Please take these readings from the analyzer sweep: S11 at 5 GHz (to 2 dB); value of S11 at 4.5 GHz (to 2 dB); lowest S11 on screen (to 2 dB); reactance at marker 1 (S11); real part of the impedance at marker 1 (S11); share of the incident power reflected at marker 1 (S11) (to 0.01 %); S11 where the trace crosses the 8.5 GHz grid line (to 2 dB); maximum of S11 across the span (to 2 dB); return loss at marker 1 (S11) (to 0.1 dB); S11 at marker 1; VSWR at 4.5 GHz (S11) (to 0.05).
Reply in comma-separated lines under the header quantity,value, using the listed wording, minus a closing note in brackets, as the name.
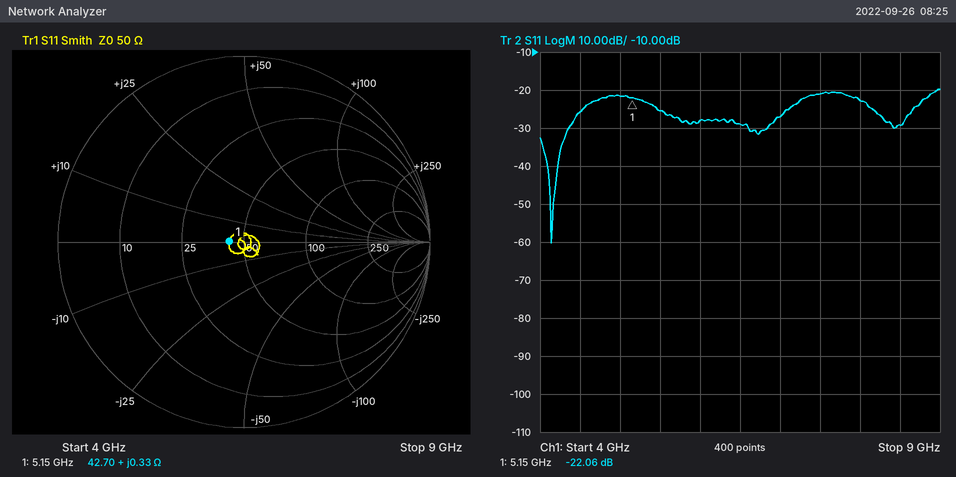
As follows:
quantity,value
S11 at 5 GHz,-22 dB
value of S11 at 4.5 GHz,-26 dB
lowest S11 on screen,-60 dB
reactance at marker 1,+0.33 Ω
real part of the impedance at marker 1,42.70 Ω
share of the incident power reflected at marker 1 (S11),0.62 %
S11 where the trace crosses the 8.5 GHz grid line,-30 dB
maximum of S11 across the span,-20 dB
return loss at marker 1 (S11),22.1 dB
S11 at marker 1,-22.06 dB
VSWR at 4.5 GHz (S11),1.10
